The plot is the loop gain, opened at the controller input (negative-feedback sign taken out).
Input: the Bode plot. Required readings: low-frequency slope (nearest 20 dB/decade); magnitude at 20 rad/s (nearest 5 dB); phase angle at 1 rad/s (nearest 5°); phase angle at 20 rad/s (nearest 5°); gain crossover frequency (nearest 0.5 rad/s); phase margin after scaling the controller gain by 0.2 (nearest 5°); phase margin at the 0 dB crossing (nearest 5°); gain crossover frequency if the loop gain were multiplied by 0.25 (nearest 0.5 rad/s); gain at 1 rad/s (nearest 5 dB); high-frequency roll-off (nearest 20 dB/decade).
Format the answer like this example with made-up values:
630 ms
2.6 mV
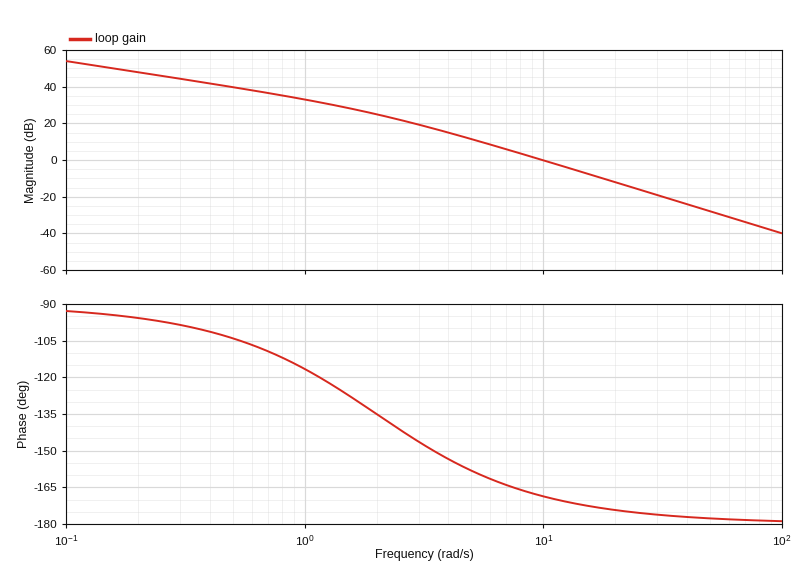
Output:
-20 dB/decade
-10 dB
-115°
-175°
10.0 rad/s
25°
10°
5.0 rad/s
35 dB
-40 dB/decade
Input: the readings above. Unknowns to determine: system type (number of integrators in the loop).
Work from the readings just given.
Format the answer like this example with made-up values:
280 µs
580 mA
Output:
1
